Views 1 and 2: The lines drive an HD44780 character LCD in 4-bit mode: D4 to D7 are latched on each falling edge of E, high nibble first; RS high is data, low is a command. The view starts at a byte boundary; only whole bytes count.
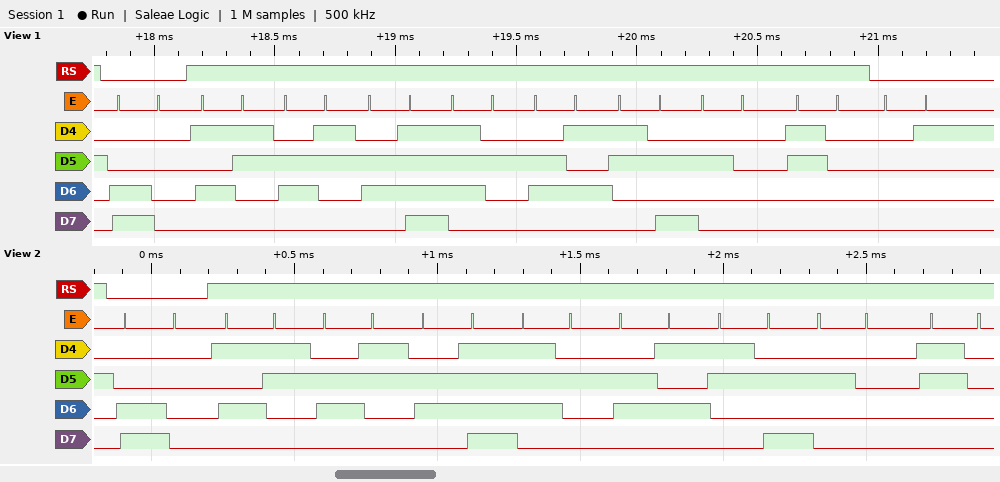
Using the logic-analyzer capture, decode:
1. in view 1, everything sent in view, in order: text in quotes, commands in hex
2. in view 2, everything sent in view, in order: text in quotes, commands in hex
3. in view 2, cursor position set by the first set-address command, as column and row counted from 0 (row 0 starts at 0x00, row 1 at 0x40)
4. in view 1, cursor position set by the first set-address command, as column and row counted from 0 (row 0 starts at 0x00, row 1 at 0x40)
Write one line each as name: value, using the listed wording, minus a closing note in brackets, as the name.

in view 1, everything sent in view, in order: text in quotes, commands in hex: 0xC0 "Score: 0" 0x01
in view 2, everything sent in view, in order: text in quotes, commands in hex: 0xC0 "Score: 0"
in view 2, cursor position set by the first set-address command, as column and row counted from 0: column 0, row 1
in view 1, cursor position set by the first set-address command, as column and row counted from 0: column 0, row 1
